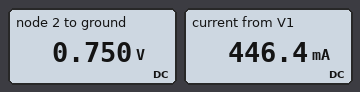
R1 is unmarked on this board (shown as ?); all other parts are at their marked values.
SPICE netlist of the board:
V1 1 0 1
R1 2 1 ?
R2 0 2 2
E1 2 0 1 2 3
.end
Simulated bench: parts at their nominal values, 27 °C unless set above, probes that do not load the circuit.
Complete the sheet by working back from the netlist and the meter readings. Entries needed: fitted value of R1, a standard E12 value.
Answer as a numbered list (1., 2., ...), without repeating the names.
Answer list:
1. 0.56 Ω
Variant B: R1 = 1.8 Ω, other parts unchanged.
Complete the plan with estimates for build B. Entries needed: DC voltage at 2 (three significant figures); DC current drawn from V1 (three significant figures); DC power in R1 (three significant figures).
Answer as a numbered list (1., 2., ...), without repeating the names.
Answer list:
1. 750 mV
2. 139 mA
3. 34.7 mW
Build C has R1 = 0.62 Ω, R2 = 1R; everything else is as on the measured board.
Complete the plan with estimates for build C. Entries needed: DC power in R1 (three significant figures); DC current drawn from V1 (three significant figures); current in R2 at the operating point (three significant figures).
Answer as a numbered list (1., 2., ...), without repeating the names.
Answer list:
1. 101 mW
2. 403 mA
3. 750 mA
